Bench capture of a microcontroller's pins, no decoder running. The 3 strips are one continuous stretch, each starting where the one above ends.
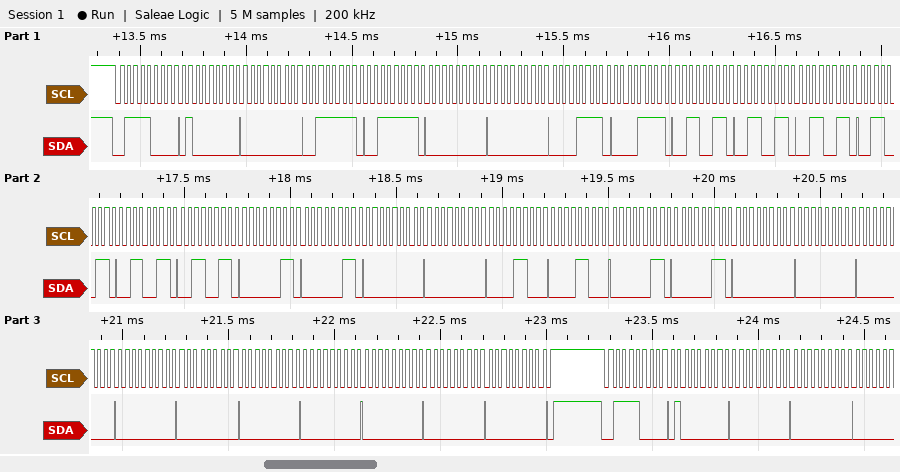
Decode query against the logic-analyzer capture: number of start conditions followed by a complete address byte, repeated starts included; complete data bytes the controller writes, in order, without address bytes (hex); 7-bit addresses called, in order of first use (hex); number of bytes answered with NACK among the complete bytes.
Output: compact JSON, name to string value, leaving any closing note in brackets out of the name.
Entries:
{"number of start conditions followed by a complete address byte, repeated starts included": "2", "complete data bytes the controller writes, in order, without address bytes": "40 00 3F 3F 00 00 0F 0F 33 33 33 33 33 33 03 03 00 00 0C 0C 03 03 00 00 00 00 00 00 00 00 00 00 40 00 00", "7-bit addresses called, in order of first use": "0x3C", "number of bytes answered with NACK among the complete bytes": "0"}
